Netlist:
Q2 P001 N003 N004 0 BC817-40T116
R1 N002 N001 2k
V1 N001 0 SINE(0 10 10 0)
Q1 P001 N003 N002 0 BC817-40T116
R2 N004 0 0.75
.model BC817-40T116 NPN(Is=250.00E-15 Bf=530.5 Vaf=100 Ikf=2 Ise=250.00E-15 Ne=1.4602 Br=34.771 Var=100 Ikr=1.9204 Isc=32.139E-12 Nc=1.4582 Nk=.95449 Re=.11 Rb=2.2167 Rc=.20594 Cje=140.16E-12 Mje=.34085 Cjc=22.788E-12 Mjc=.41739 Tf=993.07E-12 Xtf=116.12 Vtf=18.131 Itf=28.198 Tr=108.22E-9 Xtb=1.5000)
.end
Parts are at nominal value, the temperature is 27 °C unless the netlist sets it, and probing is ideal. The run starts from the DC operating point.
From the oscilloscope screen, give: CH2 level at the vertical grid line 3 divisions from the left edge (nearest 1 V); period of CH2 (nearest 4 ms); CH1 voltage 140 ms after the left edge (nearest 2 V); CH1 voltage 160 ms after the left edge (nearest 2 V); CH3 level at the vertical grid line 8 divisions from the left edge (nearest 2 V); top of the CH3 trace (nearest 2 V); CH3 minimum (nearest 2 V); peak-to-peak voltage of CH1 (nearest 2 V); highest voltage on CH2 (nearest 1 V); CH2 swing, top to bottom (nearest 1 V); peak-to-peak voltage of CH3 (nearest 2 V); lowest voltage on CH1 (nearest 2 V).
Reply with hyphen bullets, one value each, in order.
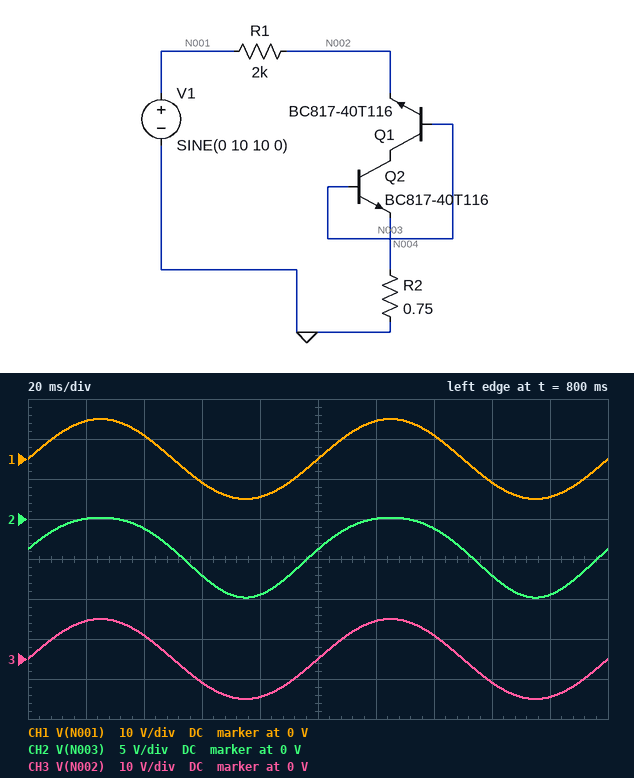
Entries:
- -7 V
- 100 ms
- 6 V
- -6 V
- -6 V
- 10 V
- -10 V
- 20 V
- 0 V
- 10 V
- 20 V
- -10 V
